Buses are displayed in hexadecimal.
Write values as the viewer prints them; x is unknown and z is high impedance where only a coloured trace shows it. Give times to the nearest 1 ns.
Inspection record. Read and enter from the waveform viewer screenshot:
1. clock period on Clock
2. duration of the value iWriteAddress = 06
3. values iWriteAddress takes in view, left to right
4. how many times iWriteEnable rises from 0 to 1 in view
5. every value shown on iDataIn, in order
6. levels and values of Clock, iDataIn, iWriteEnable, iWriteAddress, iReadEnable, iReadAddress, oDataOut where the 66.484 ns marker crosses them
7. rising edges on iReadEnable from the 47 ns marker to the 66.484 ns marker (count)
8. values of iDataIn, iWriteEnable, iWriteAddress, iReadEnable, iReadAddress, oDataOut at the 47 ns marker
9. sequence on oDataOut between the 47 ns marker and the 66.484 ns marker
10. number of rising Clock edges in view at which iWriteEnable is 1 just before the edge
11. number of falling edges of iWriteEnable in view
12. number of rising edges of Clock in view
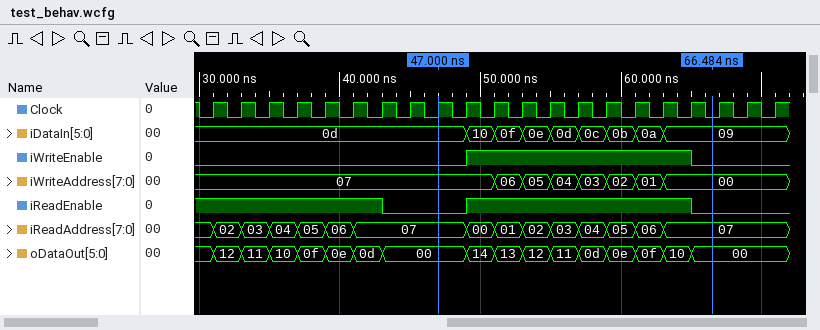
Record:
2 ns
2 ns
07, 06, 05, 04, 03, 02, 01, 00
1
0d, 10, 0f, 0e, 0d, 0c, 0b, 0a, 09
Clock=0, iDataIn=09, iWriteEnable=0, iWriteAddress=00, iReadEnable=0, iReadAddress=07, oDataOut=00
1
iDataIn=0d, iWriteEnable=0, iWriteAddress=07, iReadEnable=0, iReadAddress=07, oDataOut=00
00, 14, 13, 12, 11, 0d, 0e, 0f, 10, 00
8
1
21
